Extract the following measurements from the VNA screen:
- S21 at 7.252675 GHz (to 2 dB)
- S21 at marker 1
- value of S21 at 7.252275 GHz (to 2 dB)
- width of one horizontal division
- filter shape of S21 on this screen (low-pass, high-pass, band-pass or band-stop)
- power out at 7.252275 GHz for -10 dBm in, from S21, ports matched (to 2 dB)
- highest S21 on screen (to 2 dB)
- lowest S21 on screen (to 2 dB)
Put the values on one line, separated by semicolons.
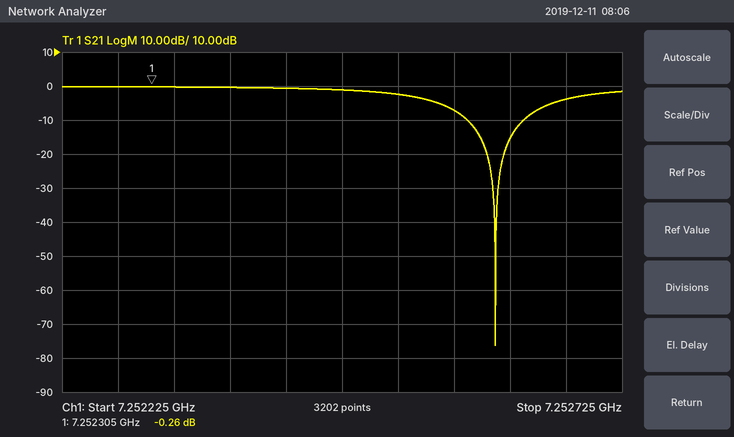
-4 dB; -0.26 dB; 0 dB; 50 kHz; band-stop; -10 dBm; 0 dB; -76 dB
